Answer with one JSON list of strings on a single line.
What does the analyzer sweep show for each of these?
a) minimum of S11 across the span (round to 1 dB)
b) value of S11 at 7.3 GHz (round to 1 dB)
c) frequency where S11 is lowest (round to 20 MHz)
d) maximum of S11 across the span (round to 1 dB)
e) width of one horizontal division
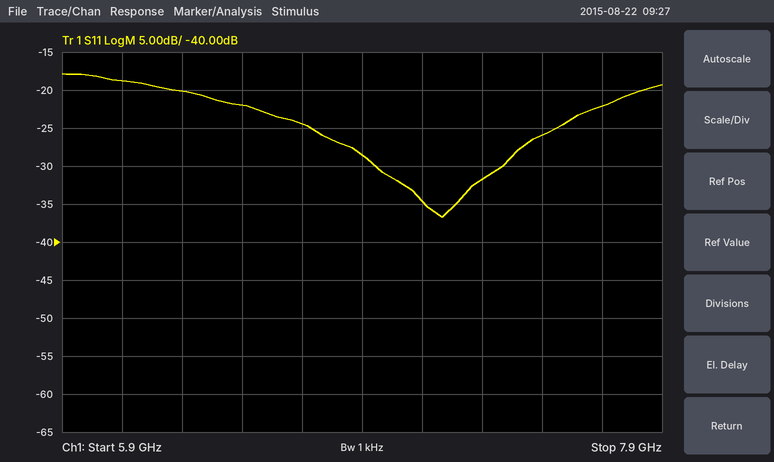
["-37 dB", "-32 dB", "7.16 GHz", "-18 dB", "200 MHz"]
